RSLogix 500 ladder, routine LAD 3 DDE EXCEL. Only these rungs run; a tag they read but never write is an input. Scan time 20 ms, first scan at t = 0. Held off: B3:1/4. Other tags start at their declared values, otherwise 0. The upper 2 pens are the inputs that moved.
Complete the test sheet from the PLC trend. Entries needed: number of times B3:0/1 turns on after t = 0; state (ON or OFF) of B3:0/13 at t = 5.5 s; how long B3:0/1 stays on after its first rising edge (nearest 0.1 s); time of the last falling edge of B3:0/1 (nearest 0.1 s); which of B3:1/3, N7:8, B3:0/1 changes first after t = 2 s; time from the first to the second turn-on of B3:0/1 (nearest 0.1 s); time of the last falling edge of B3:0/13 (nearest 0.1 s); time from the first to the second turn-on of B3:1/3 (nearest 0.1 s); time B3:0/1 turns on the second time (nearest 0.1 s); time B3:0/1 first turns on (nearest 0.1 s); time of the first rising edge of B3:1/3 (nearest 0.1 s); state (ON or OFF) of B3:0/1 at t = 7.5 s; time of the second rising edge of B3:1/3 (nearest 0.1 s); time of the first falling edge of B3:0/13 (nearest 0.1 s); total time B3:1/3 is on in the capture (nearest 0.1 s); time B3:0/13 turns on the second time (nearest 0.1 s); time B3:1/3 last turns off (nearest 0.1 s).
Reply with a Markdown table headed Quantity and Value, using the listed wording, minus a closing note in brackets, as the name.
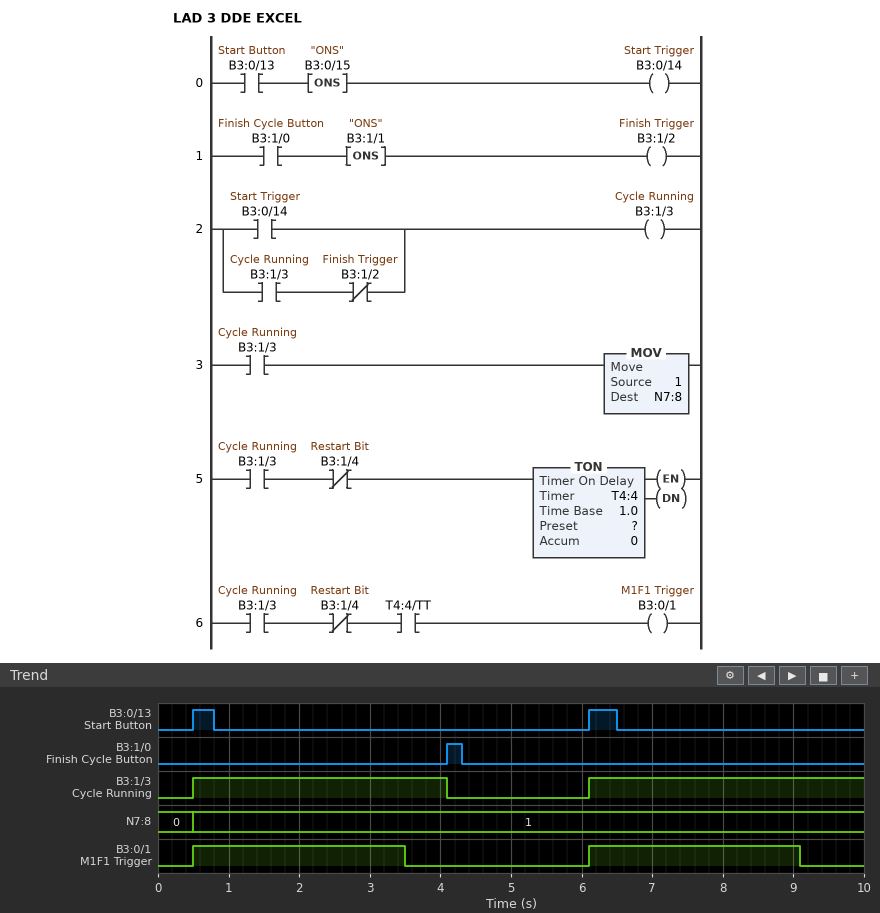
| Quantity | Value |
|---|---|
| number of times B3:0/1 turns on after t = 0 | 2 |
| state (ON or OFF) of B3:0/13 at t = 5.5 s | OFF |
| how long B3:0/1 stays on after its first rising edge | 3.0 s |
| time of the last falling edge of B3:0/1 | 9.1 s |
| which of B3:1/3, N7:8, B3:0/1 changes first after t = 2 s | B3:0/1 |
| time from the first to the second turn-on of B3:0/1 | 5.6 s |
| time of the last falling edge of B3:0/13 | 6.5 s |
| time from the first to the second turn-on of B3:1/3 | 5.6 s |
| time B3:0/1 turns on the second time | 6.1 s |
| time B3:0/1 first turns on | 0.5 s |
| time of the first rising edge of B3:1/3 | 0.5 s |
| state (ON or OFF) of B3:0/1 at t = 7.5 s | ON |
| time of the second rising edge of B3:1/3 | 6.1 s |
| time of the first falling edge of B3:0/13 | 0.8 s |
| total time B3:1/3 is on in the capture | 7.5 s |
| time B3:0/13 turns on the second time | 6.1 s |
| time B3:1/3 last turns off | 4.1 s |
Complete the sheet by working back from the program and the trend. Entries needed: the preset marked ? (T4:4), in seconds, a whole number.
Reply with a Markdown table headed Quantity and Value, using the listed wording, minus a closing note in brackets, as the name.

| Quantity | Value |
|---|---|
| the preset marked ? (T4:4), in seconds, a whole number | 3 s |
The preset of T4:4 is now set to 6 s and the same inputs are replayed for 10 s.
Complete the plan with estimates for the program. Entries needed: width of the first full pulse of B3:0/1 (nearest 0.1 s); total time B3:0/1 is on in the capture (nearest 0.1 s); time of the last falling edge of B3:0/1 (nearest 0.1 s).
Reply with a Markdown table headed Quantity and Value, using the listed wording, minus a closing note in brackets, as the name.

| Quantity | Value |
|---|---|
| width of the first full pulse of B3:0/1 | 3.6 s |
| total time B3:0/1 is on in the capture | 7.5 s |
| time of the last falling edge of B3:0/1 | 4.1 s |
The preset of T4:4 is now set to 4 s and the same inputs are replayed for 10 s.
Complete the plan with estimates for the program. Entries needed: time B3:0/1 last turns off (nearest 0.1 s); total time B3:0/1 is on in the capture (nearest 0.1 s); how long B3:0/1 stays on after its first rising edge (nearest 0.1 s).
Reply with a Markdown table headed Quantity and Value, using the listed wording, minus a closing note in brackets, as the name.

| Quantity | Value |
|---|---|
| time B3:0/1 last turns off | 4.1 s |
| total time B3:0/1 is on in the capture | 7.5 s |
| how long B3:0/1 stays on after its first rising edge | 3.6 s |
